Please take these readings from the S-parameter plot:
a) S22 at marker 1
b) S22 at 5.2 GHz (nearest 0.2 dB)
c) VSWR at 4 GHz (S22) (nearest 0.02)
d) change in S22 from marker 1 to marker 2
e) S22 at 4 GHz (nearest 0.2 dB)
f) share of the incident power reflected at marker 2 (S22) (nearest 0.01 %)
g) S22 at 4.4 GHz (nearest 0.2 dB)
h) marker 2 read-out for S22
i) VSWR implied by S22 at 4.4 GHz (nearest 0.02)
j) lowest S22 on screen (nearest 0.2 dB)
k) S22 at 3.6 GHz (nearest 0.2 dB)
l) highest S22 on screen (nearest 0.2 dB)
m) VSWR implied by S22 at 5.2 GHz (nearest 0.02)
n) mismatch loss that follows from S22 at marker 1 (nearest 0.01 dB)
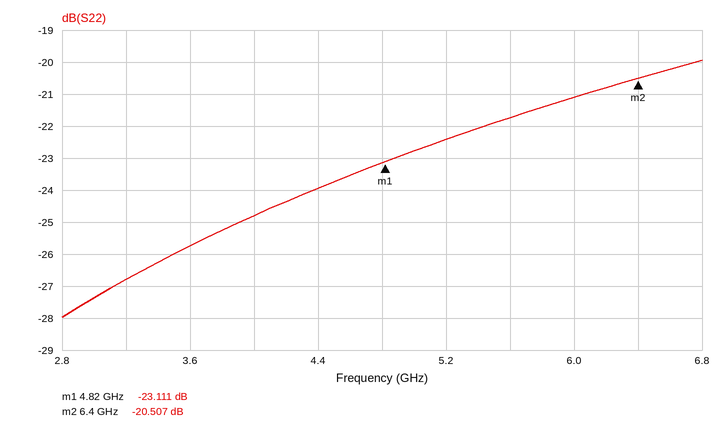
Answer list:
-23.111 dB
-22.4 dB
1.12
2.604 dB
-24.8 dB
0.89 %
-24.0 dB
-20.507 dB
1.14
-28.0 dB
-25.8 dB
-20.0 dB
1.16
0.02 dB
